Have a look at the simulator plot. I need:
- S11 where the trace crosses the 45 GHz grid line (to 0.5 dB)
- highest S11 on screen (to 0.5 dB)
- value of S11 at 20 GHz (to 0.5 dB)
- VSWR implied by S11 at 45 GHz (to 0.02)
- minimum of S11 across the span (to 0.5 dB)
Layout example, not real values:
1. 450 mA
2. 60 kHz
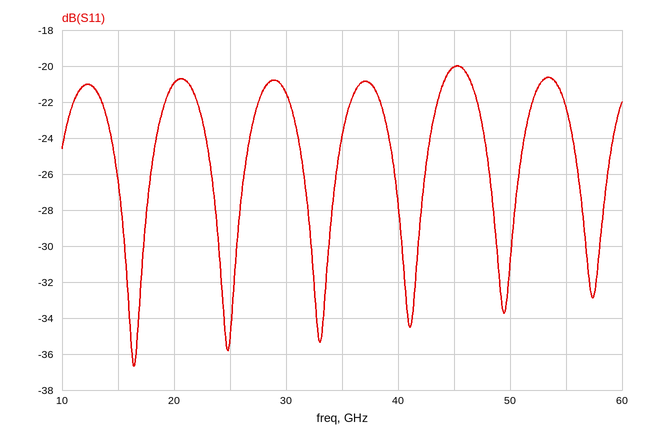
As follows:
1. -20.0 dB
2. -20.0 dB
3. -21.0 dB
4. 1.22
5. -36.5 dB
